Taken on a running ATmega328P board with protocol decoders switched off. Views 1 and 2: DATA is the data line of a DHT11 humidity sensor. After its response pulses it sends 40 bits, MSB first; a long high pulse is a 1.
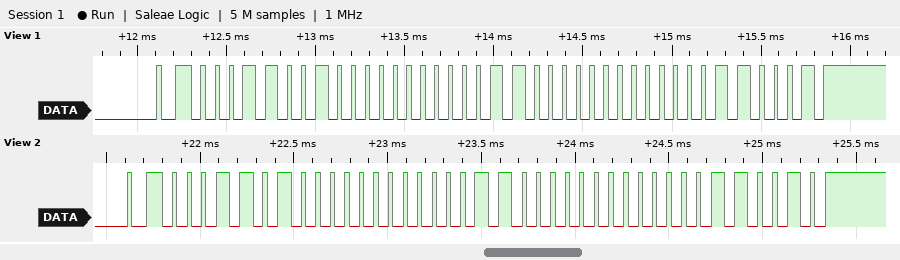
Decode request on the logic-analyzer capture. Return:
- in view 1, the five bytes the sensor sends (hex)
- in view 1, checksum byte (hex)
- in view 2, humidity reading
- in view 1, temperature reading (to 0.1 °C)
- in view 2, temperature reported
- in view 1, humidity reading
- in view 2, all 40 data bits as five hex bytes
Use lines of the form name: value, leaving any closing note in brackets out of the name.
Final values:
in view 1, the five bytes the sensor sends: 19 00 18 00 31
in view 1, checksum byte: 0x31
in view 2, humidity reading: 26 %
in view 1, temperature reading: 24.0 °C
in view 2, temperature reported: 24.0 °C
in view 1, humidity reading: 25 %
in view 2, all 40 data bits as five hex bytes: 1A 00 18 00 32
